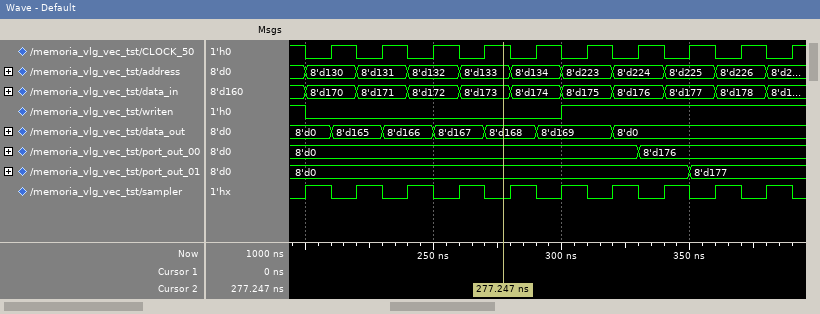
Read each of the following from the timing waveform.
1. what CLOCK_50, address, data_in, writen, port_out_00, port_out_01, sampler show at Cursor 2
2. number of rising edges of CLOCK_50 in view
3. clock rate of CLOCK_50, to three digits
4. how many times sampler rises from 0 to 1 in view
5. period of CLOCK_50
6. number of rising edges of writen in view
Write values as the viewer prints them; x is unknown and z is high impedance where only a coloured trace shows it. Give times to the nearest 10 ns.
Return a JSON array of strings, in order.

["CLOCK_50=1, address=8'd133, data_in=8'd173, writen=0, port_out_00=8'd0, port_out_01=8'd0, sampler=0", "10", "50.0 MHz", "10", "20 ns", "1"]
